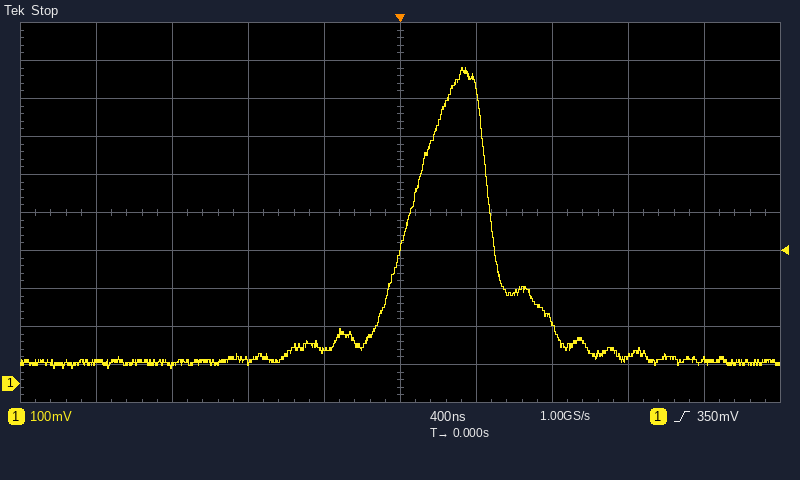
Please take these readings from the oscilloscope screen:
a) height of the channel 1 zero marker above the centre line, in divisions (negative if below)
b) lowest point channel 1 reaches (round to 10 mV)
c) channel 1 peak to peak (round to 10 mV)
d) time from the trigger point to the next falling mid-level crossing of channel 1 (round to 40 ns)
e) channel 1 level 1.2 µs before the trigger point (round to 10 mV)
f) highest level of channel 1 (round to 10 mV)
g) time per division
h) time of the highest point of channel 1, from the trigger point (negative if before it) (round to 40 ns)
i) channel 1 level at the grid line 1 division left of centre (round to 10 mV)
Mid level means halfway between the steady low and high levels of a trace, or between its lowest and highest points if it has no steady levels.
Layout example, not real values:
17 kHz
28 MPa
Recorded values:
-4.5 div
40 mV
790 mV
480 ns
50 mV
830 mV
400 ns
+320 ns
90 mV
